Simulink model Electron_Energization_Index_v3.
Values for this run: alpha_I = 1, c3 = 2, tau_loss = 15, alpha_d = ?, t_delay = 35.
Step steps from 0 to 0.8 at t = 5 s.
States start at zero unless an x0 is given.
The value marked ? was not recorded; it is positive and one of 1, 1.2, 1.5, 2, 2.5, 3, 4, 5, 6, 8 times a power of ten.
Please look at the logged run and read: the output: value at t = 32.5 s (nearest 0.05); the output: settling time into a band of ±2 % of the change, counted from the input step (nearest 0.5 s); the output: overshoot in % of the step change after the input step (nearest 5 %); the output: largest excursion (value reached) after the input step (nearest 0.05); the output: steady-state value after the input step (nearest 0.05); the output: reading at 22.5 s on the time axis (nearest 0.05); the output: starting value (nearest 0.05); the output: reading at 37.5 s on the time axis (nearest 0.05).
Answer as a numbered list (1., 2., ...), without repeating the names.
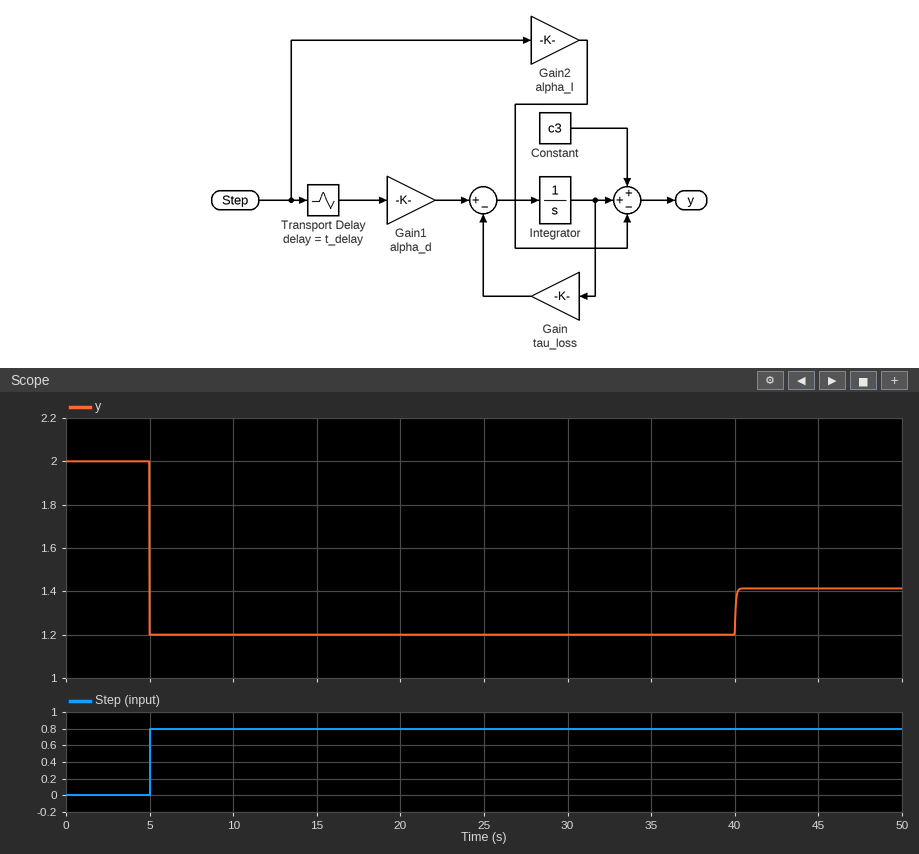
1. 1.20
2. 35.0 s
3. 35 %
4. 1.20
5. 1.40
6. 1.20
7. 2.00
8. 1.20
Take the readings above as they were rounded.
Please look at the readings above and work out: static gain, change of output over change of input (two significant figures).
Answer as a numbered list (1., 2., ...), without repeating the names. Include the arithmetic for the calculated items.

1. (1.4 - 2) / (0.8 - 0) = -0.75
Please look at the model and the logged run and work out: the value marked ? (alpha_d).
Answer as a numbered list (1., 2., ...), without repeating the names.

1. 4
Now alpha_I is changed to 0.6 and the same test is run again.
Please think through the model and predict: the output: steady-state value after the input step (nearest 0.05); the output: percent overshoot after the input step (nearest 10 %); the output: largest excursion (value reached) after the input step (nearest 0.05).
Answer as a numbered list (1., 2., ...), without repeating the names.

1. 1.75
2. 80 %
3. 1.50
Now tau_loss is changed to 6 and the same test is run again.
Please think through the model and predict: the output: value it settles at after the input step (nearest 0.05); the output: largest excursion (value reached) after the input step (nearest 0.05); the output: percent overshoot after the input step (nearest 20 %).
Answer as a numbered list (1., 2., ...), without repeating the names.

1. 1.75
2. 1.20
3. 200 %
